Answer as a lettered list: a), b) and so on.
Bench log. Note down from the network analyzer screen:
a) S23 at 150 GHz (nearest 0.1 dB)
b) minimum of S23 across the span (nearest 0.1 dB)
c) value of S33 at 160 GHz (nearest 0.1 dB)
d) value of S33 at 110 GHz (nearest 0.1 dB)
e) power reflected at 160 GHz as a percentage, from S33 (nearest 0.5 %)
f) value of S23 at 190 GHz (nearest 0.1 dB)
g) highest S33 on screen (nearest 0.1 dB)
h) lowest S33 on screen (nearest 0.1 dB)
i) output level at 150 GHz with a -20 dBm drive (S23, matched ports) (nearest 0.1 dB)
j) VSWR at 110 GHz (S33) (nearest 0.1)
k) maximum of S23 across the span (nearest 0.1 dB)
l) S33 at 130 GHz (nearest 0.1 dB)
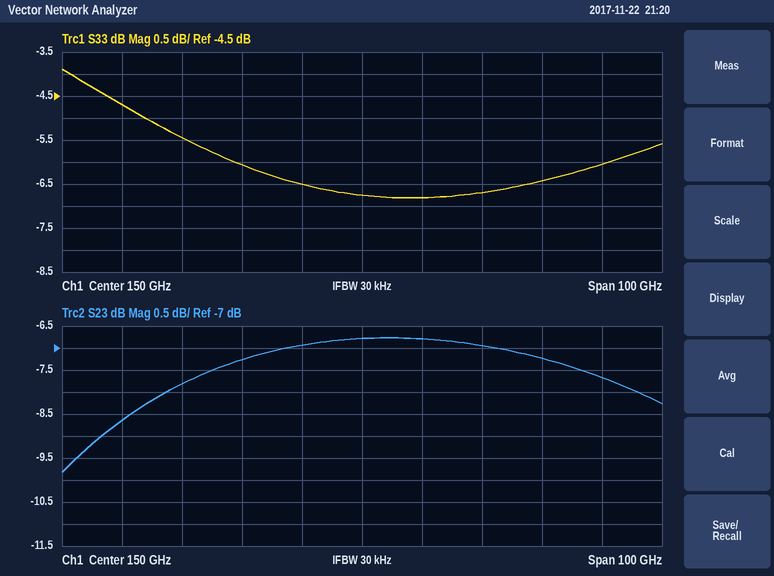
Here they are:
a) -6.8 dB
b) -9.8 dB
c) -6.8 dB
d) -4.7 dB
e) 21.0 %
f) -7.7 dB
g) -3.9 dB
h) -6.8 dB
i) -26.8 dBm
j) 3.8
k) -6.8 dB
l) -6.1 dB
